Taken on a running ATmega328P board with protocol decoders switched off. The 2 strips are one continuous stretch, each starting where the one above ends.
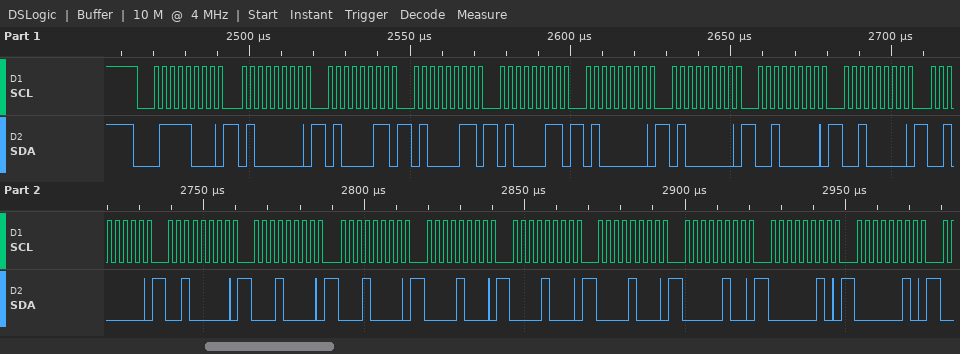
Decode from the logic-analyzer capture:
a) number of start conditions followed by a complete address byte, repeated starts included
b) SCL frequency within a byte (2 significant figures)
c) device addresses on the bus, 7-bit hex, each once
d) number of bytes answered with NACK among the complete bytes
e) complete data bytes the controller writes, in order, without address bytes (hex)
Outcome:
1
400 kHz
0x3C
0
40 43 43 43 40 40 20 20 20 20 10 10 08 08 08 04 02 02
